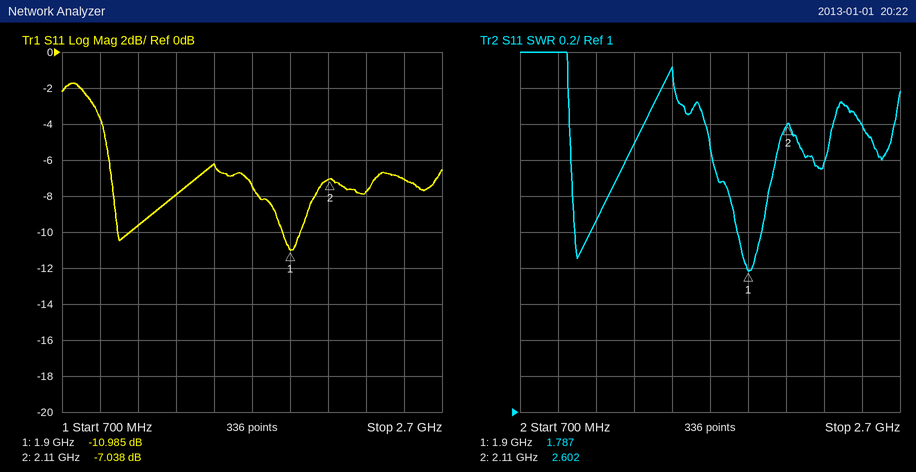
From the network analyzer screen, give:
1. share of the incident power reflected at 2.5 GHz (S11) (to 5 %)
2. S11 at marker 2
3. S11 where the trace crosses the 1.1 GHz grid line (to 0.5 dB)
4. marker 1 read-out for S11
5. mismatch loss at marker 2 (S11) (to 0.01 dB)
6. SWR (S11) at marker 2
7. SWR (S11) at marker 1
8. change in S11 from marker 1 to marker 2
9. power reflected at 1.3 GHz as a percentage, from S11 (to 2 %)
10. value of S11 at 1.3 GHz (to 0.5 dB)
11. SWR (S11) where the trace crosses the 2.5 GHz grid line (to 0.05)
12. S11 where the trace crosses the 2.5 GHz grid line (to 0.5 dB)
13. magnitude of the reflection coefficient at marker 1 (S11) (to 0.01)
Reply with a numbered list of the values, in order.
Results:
1. 20 %
2. -7.038 dB
3. -9.5 dB
4. -10.985 dB
5. 0.96 dB
6. 2.602
7. 1.787
8. 3.947 dB
9. 16 %
10. -8.0 dB
11. 2.60
12. -7.0 dB
13. 0.28
